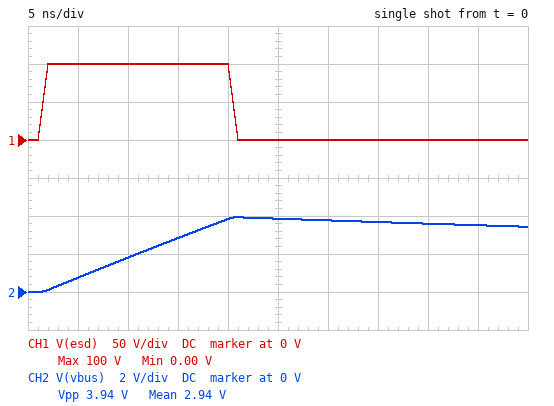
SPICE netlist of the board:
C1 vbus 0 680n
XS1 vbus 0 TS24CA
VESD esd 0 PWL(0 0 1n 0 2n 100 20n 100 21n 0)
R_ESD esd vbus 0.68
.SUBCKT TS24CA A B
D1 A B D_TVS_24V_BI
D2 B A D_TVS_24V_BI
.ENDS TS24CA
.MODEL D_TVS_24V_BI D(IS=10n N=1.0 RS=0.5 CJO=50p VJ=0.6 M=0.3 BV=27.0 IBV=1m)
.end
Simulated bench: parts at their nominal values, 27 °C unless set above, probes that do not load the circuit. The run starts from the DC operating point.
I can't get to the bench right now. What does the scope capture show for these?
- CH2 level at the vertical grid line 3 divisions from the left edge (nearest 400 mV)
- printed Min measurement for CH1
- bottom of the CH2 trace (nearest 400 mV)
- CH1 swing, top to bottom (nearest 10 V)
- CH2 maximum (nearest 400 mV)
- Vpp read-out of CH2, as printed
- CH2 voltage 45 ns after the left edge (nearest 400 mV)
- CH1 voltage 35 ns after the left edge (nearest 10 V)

2.8 V
0.00 V
0 V
100 V
4.0 V
3.94 V
3.6 V
0 V
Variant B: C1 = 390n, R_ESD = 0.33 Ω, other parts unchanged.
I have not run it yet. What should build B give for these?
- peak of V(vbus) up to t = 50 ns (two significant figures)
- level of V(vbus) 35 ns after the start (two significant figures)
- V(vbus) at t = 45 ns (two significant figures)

13 V
11 V
9.6 V
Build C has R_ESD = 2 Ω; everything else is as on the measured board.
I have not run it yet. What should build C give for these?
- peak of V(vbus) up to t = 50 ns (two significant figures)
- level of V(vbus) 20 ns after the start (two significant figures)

1.4 V
1.3 V
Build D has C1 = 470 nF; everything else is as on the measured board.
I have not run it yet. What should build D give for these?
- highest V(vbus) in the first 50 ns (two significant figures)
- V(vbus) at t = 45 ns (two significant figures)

5.6 V
4.7 V
